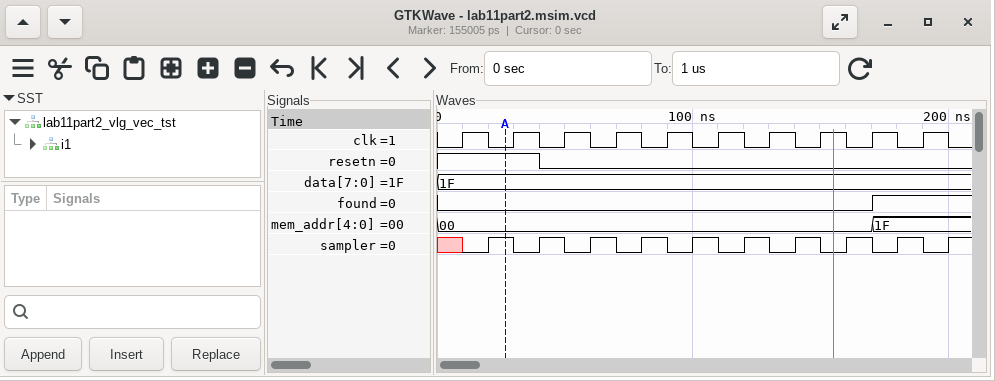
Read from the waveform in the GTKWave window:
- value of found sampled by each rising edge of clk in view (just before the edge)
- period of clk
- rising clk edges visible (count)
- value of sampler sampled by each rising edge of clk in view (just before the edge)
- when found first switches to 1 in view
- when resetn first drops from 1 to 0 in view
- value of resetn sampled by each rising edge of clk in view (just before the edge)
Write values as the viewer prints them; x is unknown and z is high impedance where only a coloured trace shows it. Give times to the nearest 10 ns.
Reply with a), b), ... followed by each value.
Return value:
a) 0 0 0 0 0 0 0 0 0 1
b) 20 ns
c) 10
d) x 1 1 1 1 1 1 1 1 1
e) 170 ns
f) 40 ns
g) 1 1 0 0 0 0 0 0 0 0
